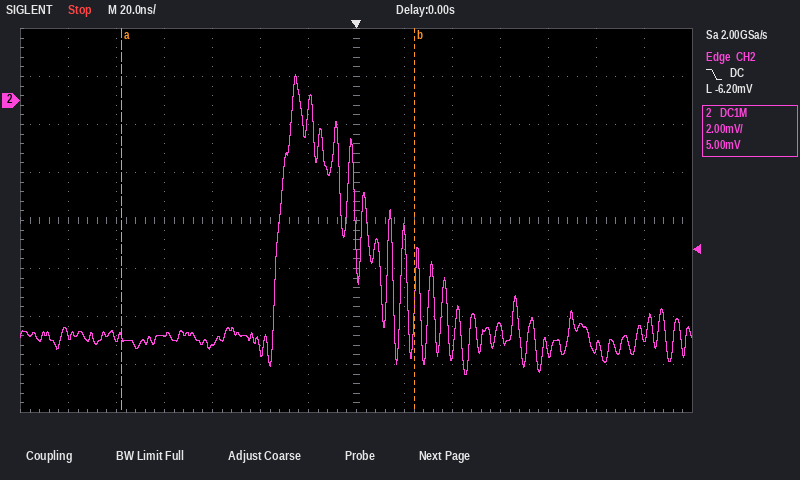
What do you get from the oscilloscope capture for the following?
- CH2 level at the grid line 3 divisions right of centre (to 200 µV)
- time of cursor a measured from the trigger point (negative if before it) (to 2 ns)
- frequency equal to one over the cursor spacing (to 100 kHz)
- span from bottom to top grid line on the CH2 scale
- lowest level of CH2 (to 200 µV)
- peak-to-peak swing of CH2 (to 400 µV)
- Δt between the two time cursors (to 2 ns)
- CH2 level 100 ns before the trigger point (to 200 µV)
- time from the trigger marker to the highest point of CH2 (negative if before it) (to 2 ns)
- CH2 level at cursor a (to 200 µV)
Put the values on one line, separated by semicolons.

-9.4 mV; -98 ns; 8.2 MHz; 16 mV; -11.4 mV; 12.4 mV; 122 ns; -10.0 mV; -26 ns; -9.8 mV
